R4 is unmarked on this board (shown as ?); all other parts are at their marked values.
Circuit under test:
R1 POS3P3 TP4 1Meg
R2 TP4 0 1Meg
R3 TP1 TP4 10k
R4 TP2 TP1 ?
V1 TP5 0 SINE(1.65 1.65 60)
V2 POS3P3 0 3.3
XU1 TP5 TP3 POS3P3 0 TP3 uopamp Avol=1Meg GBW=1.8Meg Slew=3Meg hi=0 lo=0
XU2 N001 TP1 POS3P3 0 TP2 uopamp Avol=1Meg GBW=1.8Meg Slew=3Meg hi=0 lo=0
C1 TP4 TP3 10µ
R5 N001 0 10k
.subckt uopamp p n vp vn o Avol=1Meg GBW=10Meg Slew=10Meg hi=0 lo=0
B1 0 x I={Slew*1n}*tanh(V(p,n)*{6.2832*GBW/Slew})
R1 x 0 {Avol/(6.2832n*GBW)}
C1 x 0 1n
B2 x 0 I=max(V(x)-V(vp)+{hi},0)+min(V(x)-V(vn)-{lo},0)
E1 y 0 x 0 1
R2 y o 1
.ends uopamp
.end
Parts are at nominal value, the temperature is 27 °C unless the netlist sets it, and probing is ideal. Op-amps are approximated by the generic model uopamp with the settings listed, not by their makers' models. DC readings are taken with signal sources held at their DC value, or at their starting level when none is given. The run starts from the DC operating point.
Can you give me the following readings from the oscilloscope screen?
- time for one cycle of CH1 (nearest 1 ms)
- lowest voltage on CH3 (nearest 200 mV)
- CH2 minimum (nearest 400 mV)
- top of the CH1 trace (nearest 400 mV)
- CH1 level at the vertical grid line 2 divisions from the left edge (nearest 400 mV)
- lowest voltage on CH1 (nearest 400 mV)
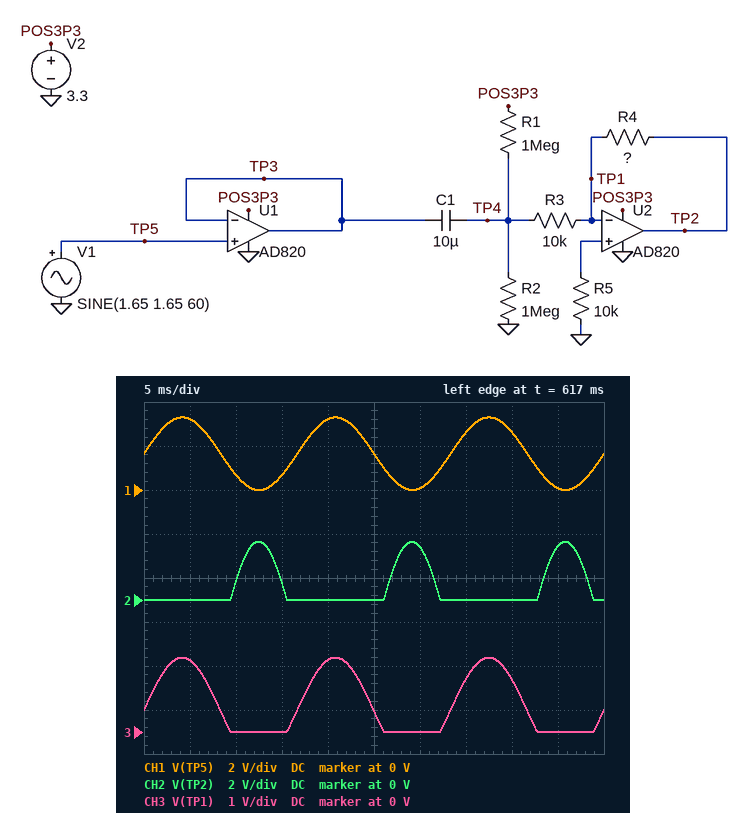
17 ms
0 V
0 V
3.2 V
800 mV
0 V
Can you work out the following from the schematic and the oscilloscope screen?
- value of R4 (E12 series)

27 kΩ
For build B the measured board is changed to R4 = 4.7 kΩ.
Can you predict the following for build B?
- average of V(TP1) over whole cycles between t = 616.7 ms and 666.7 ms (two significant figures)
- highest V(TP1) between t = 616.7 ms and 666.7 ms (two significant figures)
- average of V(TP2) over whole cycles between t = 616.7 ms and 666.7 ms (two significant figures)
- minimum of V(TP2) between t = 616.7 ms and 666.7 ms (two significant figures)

210 mV
600 mV
190 mV
-2.8 mV
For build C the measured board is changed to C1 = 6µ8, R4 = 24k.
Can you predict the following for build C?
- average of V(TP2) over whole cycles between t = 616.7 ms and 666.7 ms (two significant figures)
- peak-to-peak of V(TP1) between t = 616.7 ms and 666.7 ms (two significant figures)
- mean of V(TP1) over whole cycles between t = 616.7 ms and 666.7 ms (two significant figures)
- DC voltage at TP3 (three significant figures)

580 mV
1.6 V
630 mV
1.65 V
